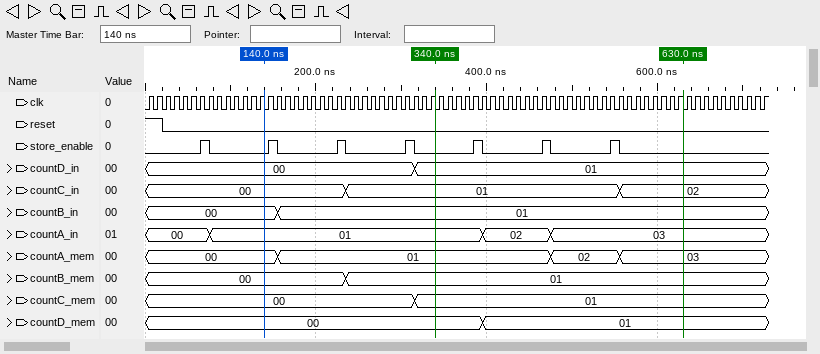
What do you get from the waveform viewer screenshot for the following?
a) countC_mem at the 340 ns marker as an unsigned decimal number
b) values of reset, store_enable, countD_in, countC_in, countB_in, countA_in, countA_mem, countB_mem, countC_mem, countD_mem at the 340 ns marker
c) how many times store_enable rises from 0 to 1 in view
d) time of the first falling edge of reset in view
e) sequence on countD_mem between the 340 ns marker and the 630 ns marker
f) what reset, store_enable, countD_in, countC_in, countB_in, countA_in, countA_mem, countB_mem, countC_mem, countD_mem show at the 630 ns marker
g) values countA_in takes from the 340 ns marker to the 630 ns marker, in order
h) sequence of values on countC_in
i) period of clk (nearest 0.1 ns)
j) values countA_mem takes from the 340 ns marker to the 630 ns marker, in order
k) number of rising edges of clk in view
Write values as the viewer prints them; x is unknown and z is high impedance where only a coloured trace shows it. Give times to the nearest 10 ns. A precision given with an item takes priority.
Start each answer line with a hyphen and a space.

- 1
- reset=0, store_enable=0, countD_in=01, countC_in=01, countB_in=01, countA_in=01, countA_mem=01, countB_mem=01, countC_mem=01, countD_mem=00
- 7
- 20 ns
- 00, 01
- reset=0, store_enable=0, countD_in=01, countC_in=02, countB_in=01, countA_in=03, countA_mem=03, countB_mem=01, countC_mem=01, countD_mem=01
- 01, 02, 03
- 00, 01, 02
- 10 ns
- 01, 02, 03
- 73
